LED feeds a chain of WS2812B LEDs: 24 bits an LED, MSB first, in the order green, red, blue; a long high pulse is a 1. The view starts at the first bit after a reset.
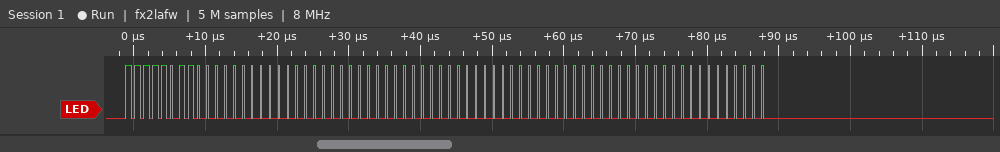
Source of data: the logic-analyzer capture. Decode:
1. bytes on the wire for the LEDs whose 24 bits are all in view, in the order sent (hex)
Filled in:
FB 00 00 00 00 00 00 00 00
